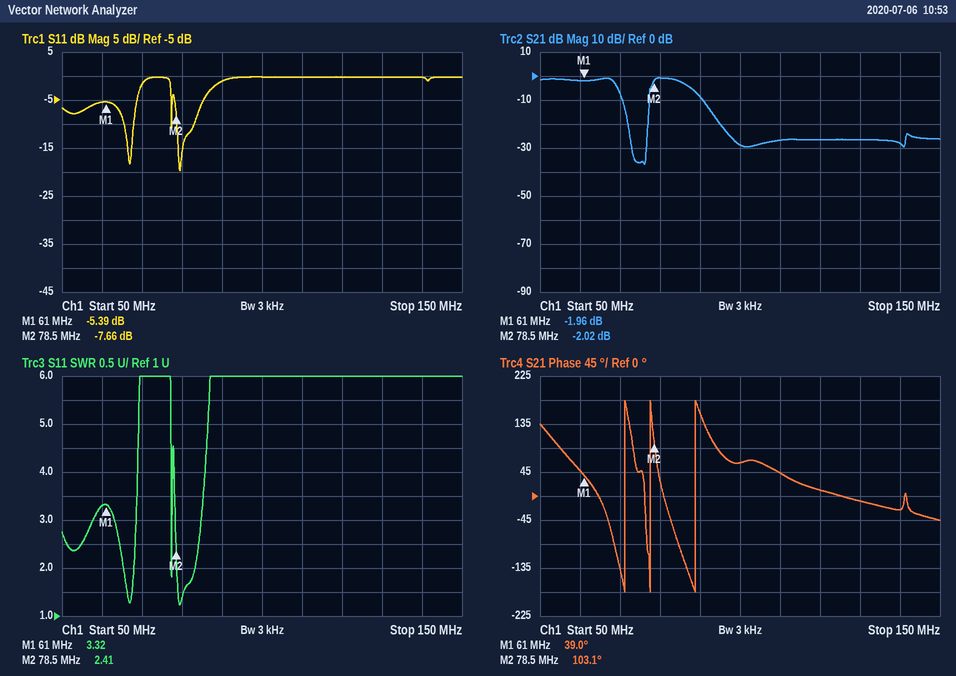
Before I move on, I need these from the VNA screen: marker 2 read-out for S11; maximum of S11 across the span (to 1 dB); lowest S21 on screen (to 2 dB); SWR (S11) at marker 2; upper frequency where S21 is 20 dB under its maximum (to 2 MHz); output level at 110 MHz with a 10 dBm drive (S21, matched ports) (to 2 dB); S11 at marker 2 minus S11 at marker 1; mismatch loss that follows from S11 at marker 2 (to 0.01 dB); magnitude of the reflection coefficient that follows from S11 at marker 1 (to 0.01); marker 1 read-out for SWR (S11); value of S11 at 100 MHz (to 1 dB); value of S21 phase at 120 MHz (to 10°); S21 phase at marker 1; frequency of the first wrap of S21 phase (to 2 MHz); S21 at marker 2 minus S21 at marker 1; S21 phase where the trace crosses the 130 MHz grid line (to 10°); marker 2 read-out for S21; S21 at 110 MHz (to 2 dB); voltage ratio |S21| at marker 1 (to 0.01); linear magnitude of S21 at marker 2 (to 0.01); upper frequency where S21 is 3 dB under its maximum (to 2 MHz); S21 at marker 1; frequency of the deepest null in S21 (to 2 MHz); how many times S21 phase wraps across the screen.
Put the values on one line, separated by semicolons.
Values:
-7.66 dB; 0 dB; -36 dB; 2.41; 96 MHz; -16 dBm; -2.27 dB; 0.82 dB; 0.54; 3.32; 0 dB; 10°; 39.0°; 72 MHz; -0.06 dB; -10°; -2.02 dB; -26 dB; 0.80; 0.79; 86 MHz; -1.96 dB; 76 MHz; 3
